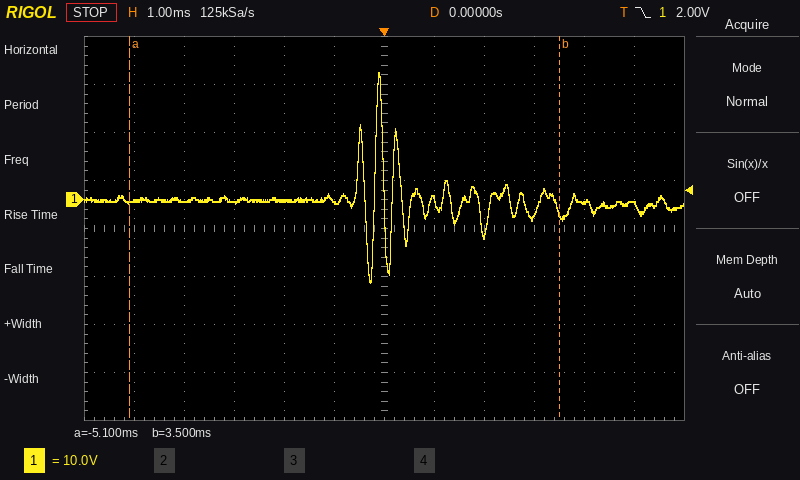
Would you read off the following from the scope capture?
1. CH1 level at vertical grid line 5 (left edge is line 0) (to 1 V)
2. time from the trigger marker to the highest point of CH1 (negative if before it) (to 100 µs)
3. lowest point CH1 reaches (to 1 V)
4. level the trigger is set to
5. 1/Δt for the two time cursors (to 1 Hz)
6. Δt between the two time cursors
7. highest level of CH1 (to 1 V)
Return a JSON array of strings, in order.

["0 V", "-100 µs", "-17 V", "2.00 V", "116 Hz", "8.6 ms", "26 V"]
